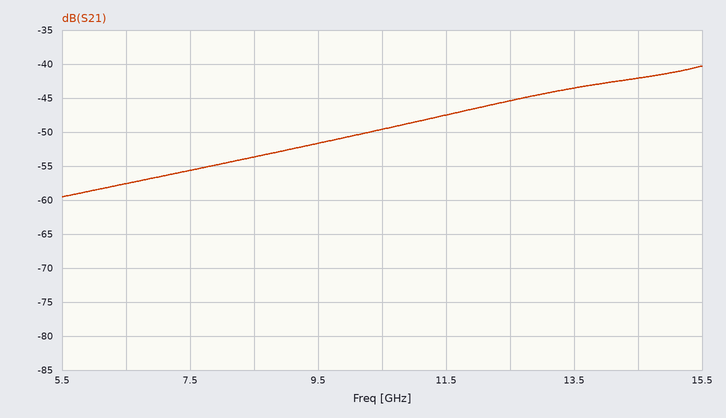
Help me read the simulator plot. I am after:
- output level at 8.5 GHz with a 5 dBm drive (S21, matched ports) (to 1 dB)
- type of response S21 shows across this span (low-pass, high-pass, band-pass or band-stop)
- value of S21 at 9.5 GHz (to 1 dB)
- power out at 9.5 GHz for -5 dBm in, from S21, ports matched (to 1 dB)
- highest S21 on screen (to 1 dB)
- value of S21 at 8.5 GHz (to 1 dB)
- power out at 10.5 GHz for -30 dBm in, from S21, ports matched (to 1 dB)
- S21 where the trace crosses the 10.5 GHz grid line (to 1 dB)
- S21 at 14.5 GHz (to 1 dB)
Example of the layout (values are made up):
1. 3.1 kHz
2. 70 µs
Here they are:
1. -49 dBm
2. high-pass
3. -52 dB
4. -57 dBm
5. -40 dB
6. -54 dB
7. -80 dBm
8. -50 dB
9. -42 dB
